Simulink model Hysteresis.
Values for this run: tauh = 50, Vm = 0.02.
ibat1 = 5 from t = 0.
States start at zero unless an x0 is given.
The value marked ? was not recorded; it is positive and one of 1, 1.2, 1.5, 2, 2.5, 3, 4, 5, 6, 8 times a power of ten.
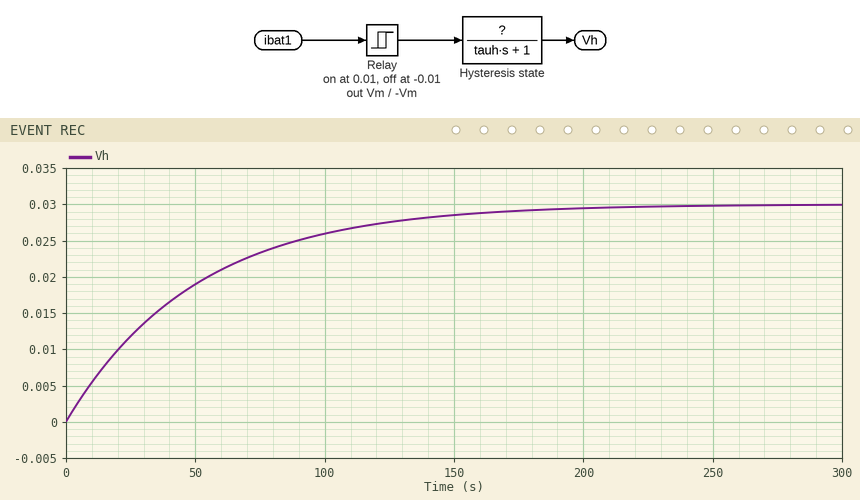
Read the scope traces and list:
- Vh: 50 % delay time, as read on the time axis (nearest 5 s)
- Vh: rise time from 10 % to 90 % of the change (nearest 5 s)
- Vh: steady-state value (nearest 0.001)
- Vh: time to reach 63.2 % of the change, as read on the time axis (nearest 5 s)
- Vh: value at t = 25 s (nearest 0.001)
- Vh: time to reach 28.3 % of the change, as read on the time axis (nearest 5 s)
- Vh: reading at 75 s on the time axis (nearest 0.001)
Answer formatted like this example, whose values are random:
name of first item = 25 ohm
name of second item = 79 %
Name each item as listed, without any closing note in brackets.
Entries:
Vh: 50 % delay time, as read on the time axis = 35 s
Vh: rise time from 10 % to 90 % of the change = 110 s
Vh: steady-state value = 0.030
Vh: time to reach 63.2 % of the change, as read on the time axis = 50 s
Vh: value at t = 25 s = 0.012
Vh: time to reach 28.3 % of the change, as read on the time axis = 15 s
Vh: reading at 75 s on the time axis = 0.023
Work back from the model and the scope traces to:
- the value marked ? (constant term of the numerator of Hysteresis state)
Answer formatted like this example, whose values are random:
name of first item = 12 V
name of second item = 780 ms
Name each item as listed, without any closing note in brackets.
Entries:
the value marked ? = 1.5
